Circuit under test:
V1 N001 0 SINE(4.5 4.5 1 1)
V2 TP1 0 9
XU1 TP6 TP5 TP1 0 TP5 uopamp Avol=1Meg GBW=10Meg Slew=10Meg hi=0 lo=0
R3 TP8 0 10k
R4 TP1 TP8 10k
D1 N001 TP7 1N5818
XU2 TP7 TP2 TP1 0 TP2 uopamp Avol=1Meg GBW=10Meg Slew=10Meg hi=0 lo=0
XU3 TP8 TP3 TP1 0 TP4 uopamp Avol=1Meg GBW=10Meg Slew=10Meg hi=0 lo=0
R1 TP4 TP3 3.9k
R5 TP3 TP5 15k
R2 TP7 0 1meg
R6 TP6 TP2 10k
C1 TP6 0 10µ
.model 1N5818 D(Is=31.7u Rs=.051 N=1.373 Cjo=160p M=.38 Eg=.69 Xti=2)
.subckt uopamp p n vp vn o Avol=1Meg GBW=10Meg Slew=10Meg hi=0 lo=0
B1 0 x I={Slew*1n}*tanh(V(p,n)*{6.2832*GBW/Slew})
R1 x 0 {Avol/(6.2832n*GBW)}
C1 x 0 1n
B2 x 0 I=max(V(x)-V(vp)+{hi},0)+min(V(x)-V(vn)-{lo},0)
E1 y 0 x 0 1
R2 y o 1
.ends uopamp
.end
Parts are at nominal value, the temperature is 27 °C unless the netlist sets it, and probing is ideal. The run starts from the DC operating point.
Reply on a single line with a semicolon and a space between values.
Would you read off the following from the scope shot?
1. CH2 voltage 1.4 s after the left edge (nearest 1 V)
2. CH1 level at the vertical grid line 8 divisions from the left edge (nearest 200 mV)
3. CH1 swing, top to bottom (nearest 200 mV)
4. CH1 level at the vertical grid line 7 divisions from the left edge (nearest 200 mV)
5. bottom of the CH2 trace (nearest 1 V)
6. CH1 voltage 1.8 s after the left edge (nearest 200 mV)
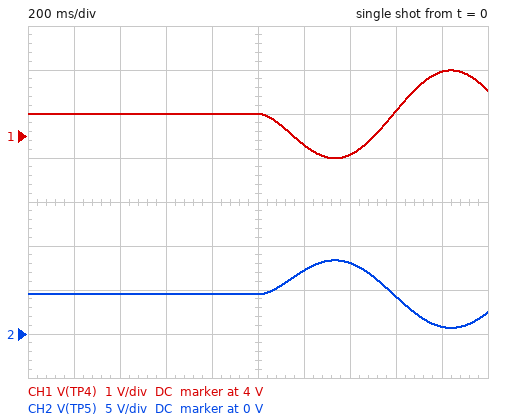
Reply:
8 V; 4.6 V; 2.0 V; 3.6 V; 1 V; 5.4 V
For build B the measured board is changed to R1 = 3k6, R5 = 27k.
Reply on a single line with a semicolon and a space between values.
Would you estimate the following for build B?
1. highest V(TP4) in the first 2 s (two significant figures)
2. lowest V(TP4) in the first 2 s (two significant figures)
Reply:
5.0 V; 4.0 V
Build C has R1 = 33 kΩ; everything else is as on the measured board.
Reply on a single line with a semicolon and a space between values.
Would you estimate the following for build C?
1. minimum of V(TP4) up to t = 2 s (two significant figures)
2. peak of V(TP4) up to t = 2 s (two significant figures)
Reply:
-9.8 mV; 9.0 V
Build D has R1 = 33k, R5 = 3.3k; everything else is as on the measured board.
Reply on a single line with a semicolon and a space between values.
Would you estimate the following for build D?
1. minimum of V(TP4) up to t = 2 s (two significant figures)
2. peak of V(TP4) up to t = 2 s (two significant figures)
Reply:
-9.8 mV; 9.0 V
